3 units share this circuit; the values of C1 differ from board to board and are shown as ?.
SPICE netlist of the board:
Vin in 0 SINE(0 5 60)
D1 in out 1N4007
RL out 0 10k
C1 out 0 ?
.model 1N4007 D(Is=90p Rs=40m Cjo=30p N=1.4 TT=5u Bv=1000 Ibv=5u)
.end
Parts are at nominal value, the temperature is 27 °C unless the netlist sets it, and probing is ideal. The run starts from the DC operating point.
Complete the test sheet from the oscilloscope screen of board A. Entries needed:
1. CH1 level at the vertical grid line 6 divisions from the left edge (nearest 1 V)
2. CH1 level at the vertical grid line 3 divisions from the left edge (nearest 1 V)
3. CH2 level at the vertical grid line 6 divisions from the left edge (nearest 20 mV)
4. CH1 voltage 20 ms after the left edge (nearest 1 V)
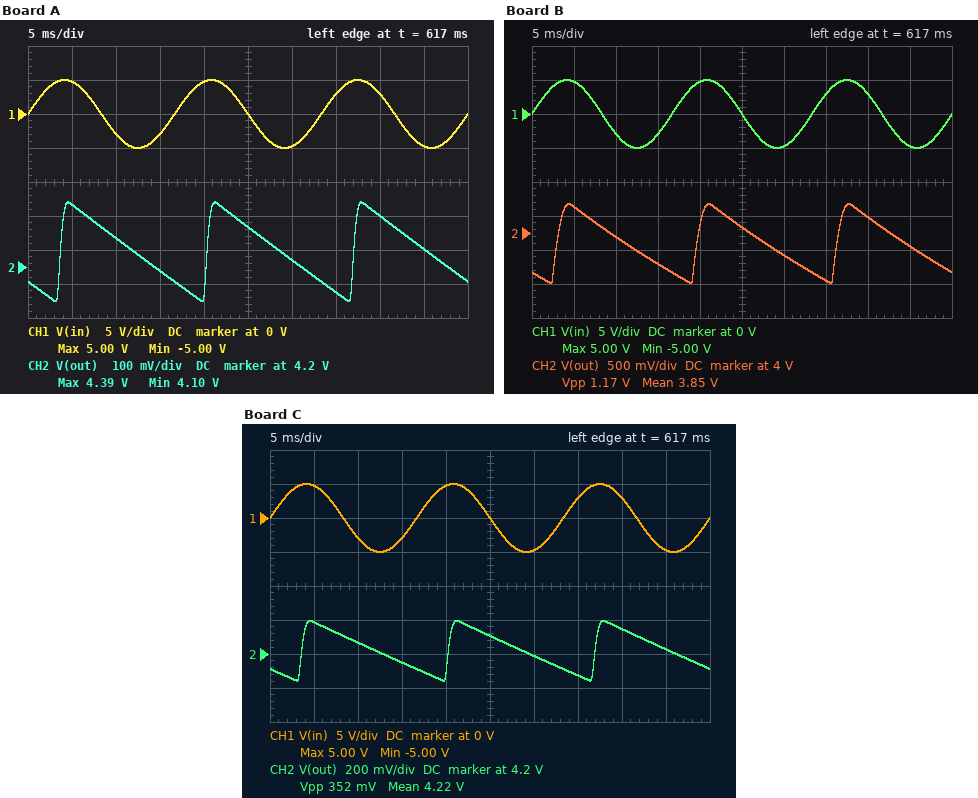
-5 V
-3 V
4.22 V
5 V
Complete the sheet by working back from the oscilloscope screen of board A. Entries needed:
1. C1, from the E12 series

22 µF
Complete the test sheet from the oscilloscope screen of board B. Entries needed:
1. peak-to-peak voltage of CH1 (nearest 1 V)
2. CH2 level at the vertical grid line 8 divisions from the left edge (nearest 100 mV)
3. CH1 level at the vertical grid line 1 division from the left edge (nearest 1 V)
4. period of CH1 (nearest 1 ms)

10 V
4.2 V
5 V
17 ms
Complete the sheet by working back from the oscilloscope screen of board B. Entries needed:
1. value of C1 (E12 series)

4.7 µF
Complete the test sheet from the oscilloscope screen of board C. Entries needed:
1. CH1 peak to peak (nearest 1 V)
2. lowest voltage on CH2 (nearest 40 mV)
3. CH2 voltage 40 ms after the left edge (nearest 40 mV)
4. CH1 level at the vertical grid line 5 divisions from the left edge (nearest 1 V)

10 V
4.04 V
4.36 V
0 V
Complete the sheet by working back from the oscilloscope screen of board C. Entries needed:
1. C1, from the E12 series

18 µF
